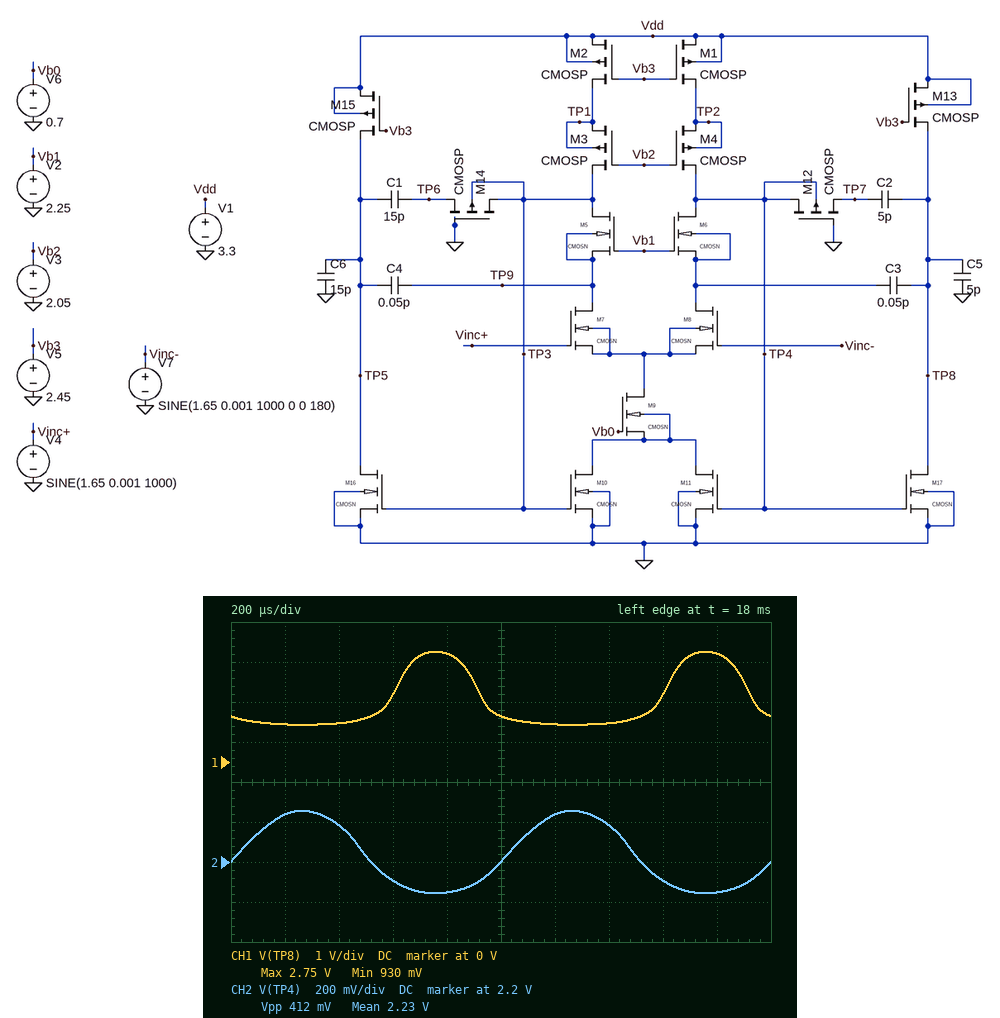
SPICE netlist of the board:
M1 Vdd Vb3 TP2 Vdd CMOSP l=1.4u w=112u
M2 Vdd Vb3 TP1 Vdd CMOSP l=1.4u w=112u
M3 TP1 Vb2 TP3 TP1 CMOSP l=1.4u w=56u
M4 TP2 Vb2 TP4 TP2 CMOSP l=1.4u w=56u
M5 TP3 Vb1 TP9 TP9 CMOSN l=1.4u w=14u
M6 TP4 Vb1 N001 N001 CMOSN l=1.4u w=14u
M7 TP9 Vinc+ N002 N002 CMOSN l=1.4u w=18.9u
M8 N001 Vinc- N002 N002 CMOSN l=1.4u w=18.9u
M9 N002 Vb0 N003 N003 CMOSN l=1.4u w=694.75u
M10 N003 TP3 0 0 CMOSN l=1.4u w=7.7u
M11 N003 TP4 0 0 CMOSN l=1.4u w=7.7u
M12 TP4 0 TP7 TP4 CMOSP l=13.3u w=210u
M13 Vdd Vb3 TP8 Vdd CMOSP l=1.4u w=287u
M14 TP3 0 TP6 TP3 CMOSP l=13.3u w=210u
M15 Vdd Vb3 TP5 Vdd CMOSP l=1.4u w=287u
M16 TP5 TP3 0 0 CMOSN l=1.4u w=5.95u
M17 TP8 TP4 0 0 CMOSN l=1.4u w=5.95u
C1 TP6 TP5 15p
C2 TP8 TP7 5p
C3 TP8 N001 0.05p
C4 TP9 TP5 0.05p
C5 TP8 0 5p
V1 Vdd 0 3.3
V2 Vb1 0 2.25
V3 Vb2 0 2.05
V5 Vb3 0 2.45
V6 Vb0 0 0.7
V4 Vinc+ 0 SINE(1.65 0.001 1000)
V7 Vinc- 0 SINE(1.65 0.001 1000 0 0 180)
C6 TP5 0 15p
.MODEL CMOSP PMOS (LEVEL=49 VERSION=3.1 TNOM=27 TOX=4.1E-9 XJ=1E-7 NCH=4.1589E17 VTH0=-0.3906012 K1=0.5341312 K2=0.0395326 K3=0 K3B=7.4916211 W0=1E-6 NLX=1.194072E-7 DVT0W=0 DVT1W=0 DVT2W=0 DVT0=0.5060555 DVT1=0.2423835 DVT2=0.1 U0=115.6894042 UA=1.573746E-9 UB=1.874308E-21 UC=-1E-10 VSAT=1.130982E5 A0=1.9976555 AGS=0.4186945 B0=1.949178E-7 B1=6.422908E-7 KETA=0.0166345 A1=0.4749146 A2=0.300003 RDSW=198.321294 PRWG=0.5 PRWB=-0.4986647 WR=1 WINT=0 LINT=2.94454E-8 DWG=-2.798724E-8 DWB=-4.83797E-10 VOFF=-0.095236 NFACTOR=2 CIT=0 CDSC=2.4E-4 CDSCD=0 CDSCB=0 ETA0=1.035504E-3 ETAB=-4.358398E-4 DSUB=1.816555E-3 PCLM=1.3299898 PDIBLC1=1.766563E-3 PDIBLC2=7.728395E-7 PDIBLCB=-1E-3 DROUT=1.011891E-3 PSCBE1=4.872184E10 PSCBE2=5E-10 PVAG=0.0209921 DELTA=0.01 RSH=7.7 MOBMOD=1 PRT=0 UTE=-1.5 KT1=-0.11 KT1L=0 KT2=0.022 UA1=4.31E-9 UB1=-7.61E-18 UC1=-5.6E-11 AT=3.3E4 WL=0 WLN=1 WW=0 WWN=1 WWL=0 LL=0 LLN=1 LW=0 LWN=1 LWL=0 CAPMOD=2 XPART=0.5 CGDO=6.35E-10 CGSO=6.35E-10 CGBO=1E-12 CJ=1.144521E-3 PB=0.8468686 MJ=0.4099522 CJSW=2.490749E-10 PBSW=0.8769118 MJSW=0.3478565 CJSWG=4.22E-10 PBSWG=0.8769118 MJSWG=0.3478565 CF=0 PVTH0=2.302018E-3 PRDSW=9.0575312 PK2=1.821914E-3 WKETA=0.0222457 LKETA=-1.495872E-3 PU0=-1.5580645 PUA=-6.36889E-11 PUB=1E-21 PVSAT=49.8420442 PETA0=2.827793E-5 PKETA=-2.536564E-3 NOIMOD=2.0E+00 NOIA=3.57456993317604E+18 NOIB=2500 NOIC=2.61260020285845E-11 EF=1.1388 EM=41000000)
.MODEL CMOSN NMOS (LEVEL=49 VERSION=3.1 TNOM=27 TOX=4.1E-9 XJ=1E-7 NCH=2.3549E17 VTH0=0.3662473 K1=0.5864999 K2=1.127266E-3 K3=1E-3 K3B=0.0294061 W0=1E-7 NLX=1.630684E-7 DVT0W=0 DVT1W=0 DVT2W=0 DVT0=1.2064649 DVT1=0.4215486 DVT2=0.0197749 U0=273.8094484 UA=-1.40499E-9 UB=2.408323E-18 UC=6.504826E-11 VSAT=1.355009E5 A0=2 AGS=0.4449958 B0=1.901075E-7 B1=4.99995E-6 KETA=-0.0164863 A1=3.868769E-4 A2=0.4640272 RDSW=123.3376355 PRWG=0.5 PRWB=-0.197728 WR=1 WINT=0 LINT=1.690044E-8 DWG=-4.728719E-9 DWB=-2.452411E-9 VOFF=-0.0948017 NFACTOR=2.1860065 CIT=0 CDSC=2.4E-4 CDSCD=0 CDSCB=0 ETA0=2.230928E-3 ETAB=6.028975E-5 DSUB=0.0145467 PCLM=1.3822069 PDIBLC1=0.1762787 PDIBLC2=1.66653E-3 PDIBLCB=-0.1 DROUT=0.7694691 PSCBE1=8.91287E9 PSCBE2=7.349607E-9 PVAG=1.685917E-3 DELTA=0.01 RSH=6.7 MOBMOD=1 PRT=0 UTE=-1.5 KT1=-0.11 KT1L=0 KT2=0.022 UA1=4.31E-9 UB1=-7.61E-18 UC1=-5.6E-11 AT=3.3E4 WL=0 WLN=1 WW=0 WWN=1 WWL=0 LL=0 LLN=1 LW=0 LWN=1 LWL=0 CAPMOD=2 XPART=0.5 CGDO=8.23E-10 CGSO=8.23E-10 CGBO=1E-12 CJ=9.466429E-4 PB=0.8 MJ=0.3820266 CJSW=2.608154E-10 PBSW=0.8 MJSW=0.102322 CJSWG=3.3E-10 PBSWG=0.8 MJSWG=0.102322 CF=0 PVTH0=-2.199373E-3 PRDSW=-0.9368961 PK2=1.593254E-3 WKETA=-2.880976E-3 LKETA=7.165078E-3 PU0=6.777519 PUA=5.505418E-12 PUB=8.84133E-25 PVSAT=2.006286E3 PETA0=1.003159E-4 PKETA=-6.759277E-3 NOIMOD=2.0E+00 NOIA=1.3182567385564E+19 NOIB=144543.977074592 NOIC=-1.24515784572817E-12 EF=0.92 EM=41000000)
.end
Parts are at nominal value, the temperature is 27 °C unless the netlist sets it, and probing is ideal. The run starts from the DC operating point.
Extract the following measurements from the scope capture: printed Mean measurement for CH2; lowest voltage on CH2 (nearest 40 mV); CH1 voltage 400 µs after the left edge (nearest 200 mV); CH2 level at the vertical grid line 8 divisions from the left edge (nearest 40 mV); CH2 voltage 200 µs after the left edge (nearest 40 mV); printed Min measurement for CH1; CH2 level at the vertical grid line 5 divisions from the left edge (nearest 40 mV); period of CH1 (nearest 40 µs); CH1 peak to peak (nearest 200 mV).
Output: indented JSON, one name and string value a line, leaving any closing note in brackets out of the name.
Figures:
{
  "printed Mean measurement for CH2": "2.23 V",
  "lowest voltage on CH2": "2.04 V",
  "CH1 voltage 400 µs after the left edge": "1.0 V",
  "CH2 level at the vertical grid line 8 divisions from the left edge": "2.12 V",
  "CH2 voltage 200 µs after the left edge": "2.44 V",
  "printed Min measurement for CH1": "930 mV",
  "CH2 level at the vertical grid line 5 divisions from the left edge": "2.20 V",
  "period of CH1": "1.00 ms",
  "CH1 peak to peak": "1.8 V"
}
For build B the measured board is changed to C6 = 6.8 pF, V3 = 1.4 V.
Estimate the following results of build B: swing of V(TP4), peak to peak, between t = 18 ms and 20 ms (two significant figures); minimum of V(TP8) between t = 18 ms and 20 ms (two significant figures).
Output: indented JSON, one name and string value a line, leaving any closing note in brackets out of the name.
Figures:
{
  "swing of V(TP4), peak to peak, between t = 18 ms and 20 ms": "7.5 mV",
  "minimum of V(TP8) between t = 18 ms and 20 ms": "830 mV"
}
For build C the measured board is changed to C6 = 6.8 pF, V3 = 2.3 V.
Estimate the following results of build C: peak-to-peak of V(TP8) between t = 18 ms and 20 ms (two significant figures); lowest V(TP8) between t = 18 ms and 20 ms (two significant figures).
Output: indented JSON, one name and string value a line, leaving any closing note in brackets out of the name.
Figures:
{
  "peak-to-peak of V(TP8) between t = 18 ms and 20 ms": "2.2 mV",
  "lowest V(TP8) between t = 18 ms and 20 ms": "3.2 V"
}
